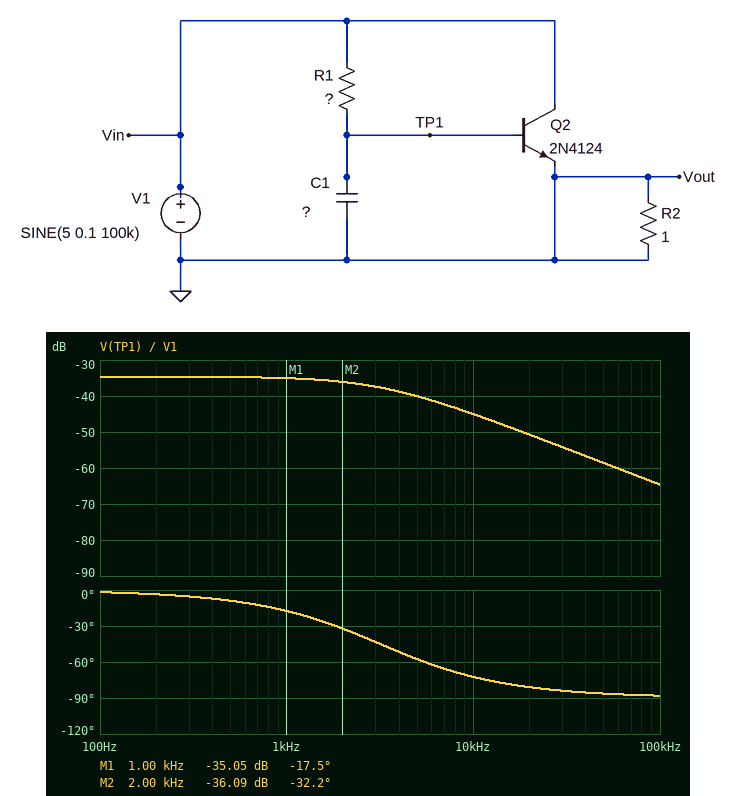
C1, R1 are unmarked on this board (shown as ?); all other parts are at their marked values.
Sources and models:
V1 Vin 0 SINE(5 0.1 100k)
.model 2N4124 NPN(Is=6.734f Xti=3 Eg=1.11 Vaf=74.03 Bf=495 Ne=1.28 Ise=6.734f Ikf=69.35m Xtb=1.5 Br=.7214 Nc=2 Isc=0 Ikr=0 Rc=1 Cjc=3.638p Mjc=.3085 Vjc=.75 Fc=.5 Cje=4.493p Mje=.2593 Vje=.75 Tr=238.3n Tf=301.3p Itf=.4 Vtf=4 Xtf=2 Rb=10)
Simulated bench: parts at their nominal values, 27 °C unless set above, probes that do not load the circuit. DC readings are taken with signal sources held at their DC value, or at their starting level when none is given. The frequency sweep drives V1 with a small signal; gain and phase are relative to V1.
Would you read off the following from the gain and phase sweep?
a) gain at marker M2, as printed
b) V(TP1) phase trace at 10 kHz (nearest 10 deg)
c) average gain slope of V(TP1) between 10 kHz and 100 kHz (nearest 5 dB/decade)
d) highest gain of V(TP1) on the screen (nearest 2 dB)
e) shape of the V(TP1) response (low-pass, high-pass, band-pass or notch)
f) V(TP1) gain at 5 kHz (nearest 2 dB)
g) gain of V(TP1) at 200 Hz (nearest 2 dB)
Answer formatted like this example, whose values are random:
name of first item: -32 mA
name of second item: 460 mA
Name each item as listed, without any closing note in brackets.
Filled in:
gain at marker M2, as printed: -36.09 dB
V(TP1) phase trace at 10 kHz: -70 deg
average gain slope of V(TP1) between 10 kHz and 100 kHz: -20 dB/decade
highest gain of V(TP1) on the screen: -34 dB
shape of the V(TP1) response: low-pass
V(TP1) gain at 5 kHz: -40 dB
gain of V(TP1) at 200 Hz: -34 dB
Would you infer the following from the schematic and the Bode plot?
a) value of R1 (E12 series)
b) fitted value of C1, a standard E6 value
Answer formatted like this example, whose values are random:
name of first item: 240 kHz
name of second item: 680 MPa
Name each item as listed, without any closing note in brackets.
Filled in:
value of R1: 820 Ω
fitted value of C1, a standard E6 value: 3.3 µF
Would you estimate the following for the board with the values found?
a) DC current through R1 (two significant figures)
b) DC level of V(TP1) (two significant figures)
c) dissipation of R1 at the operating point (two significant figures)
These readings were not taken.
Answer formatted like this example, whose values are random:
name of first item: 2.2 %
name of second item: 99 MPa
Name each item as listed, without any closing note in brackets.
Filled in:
DC current through R1: 5.0 mA
DC level of V(TP1): 910 mV
dissipation of R1 at the operating point: 20 mW
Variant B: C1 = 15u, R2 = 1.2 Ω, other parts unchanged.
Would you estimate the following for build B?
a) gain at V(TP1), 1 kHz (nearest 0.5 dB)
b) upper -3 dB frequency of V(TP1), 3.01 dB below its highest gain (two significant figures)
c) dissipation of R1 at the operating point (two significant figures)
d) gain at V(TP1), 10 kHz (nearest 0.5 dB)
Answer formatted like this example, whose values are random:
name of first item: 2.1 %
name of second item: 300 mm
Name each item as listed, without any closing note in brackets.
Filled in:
gain at V(TP1), 1 kHz: -39.5 dB
upper -3 dB frequency of V(TP1), 3.01 dB below its highest gain: 700 Hz
dissipation of R1 at the operating point: 20 mW
gain at V(TP1), 10 kHz: -58.0 dB
